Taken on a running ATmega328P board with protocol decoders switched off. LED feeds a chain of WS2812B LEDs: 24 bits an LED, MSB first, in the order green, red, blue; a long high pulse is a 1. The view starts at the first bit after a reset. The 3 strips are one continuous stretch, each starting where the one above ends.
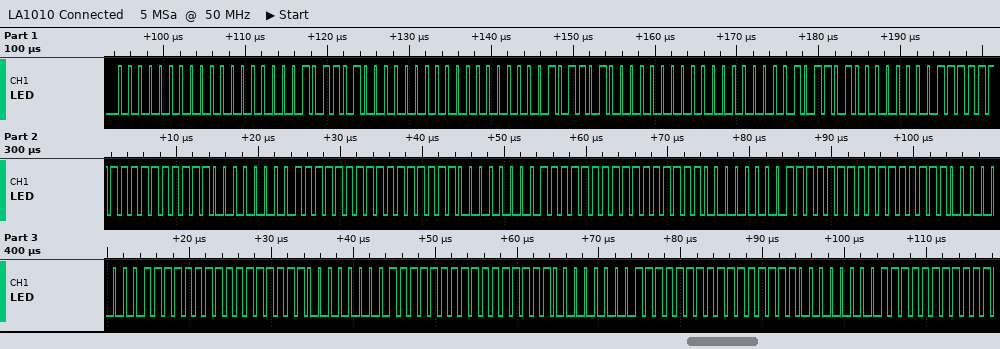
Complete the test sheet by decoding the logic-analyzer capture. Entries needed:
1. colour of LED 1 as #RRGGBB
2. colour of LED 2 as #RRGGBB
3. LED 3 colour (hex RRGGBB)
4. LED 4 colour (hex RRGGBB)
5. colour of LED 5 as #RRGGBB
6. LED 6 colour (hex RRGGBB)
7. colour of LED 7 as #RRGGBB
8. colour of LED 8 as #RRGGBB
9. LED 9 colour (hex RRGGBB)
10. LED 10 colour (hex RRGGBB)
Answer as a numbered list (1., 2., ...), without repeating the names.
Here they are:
1. #00002D
2. #00002D
3. #00002D
4. #FF00FF
5. #FF00FF
6. #FF00FF
7. #FF00FF
8. #FF00FF
9. #FF00FF
10. #FF00FF
